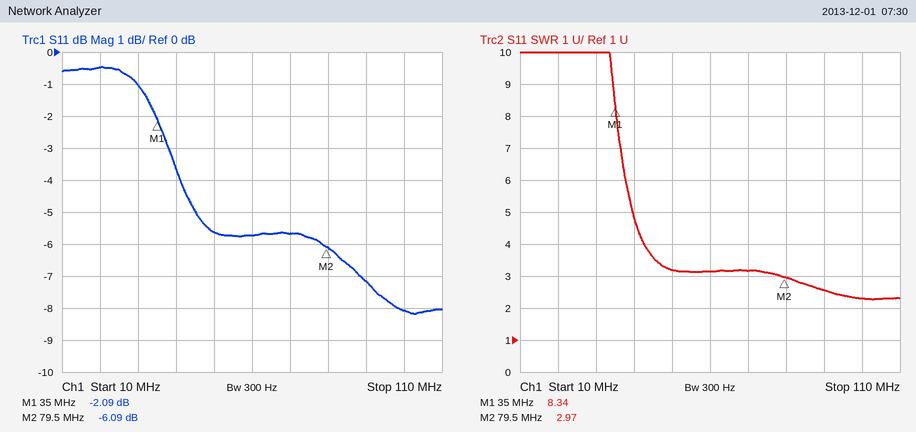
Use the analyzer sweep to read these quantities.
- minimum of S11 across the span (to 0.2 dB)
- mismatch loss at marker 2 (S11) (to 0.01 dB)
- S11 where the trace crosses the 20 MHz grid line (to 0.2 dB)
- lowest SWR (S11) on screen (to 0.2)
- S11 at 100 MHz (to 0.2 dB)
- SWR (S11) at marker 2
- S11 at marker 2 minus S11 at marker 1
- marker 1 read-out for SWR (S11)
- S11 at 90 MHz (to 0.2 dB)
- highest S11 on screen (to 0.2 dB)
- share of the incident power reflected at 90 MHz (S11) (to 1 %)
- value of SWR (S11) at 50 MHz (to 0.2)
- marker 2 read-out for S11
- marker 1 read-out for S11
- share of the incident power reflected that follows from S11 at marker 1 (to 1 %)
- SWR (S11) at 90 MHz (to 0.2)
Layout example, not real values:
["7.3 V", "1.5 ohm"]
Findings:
["-8.2 dB", "1.23 dB", "-0.4 dB", "2.2", "-8.0 dB", "2.97", "-4.00 dB", "8.34", "-7.2 dB", "-0.4 dB", "19 %", "3.2", "-6.09 dB", "-2.09 dB", "62 %", "2.6"]
